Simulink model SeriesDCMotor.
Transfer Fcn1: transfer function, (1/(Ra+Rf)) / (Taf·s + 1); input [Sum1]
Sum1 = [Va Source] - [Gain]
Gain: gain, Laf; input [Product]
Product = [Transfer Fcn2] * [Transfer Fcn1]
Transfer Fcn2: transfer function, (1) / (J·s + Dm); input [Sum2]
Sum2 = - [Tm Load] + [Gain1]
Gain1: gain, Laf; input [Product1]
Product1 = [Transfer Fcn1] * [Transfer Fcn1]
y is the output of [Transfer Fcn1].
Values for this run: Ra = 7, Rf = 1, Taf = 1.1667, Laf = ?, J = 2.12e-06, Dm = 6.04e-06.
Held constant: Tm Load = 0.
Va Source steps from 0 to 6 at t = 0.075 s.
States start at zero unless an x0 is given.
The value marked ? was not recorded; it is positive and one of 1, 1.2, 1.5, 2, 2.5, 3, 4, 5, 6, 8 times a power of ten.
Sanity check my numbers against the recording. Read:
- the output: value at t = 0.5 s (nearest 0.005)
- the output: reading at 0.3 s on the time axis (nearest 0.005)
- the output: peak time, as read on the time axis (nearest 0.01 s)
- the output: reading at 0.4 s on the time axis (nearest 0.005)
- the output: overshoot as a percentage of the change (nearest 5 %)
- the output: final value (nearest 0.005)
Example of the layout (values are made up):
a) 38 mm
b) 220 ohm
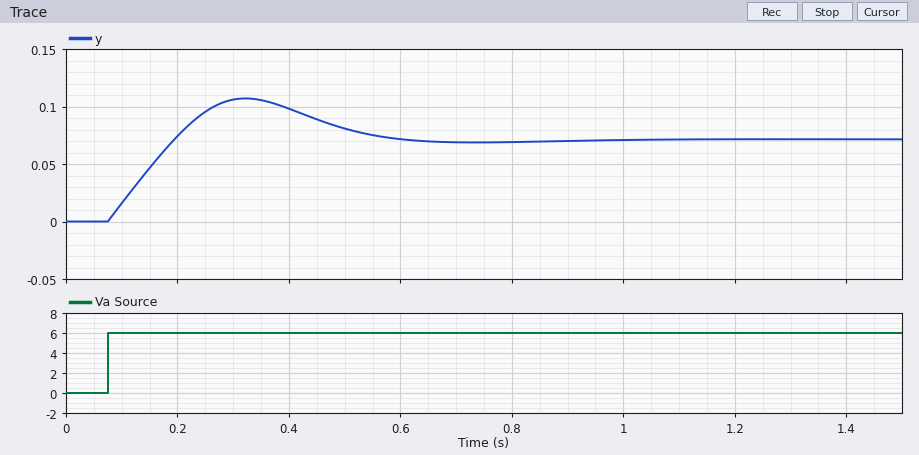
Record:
a) 0.080
b) 0.105
c) 0.32 s
d) 0.100
e) 50 %
f) 0.070
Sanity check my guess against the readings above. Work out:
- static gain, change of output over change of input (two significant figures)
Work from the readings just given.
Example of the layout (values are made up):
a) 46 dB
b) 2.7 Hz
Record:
a) 0.012
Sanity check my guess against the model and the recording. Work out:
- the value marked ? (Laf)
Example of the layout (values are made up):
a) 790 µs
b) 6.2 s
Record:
a) 0.3
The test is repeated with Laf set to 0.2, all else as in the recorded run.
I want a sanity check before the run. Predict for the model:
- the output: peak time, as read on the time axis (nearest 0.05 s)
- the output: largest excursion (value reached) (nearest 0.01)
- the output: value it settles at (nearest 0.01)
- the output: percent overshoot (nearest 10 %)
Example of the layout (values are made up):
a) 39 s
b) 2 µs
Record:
a) 0.40 s
b) 0.13
c) 0.09
d) 40 %
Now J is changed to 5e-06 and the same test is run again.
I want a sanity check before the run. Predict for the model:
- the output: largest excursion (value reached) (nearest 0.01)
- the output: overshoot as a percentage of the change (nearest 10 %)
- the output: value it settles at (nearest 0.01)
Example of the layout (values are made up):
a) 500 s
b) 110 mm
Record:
a) 0.13
b) 80 %
c) 0.07
